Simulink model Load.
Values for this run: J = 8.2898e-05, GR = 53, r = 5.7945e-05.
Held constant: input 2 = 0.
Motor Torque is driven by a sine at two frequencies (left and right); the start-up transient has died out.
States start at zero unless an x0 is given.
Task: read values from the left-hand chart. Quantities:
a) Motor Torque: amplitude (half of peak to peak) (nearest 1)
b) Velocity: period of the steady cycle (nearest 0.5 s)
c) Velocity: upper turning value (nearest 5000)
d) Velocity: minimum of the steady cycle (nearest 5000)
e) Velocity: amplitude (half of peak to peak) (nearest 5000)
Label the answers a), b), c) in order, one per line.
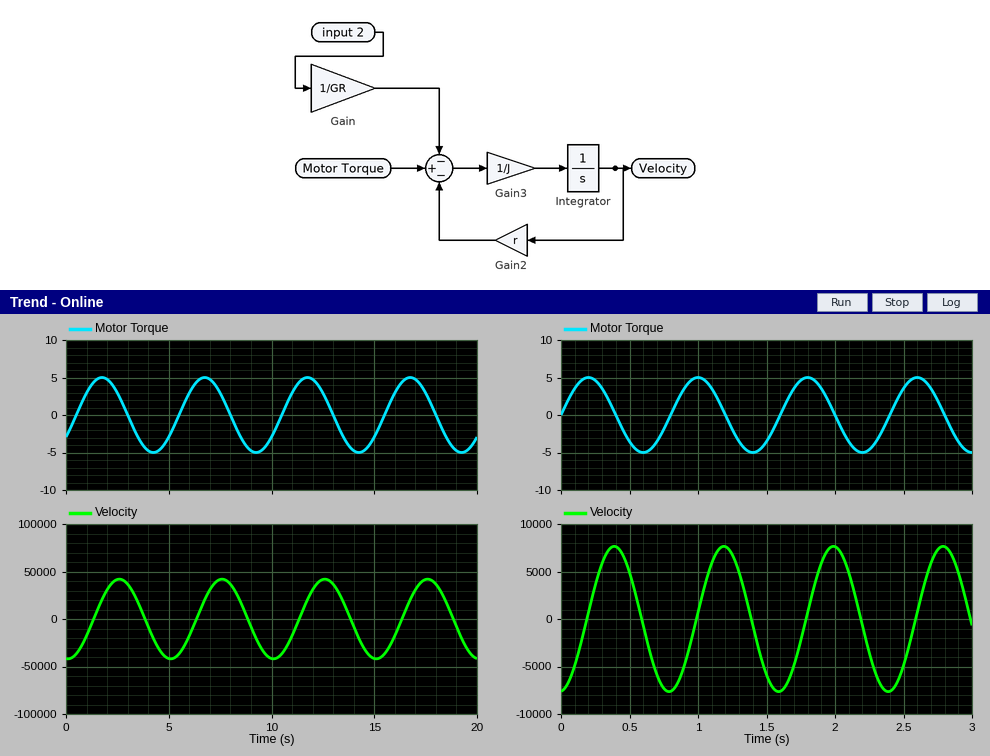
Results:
a) 5
b) 5.0 s
c) 40000
d) -40000
e) 40000
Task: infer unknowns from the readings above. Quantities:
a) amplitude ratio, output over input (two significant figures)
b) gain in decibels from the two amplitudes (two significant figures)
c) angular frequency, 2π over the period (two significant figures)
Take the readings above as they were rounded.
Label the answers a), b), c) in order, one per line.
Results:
a) 8000
b) 78 dB
c) 1.3 rad/s
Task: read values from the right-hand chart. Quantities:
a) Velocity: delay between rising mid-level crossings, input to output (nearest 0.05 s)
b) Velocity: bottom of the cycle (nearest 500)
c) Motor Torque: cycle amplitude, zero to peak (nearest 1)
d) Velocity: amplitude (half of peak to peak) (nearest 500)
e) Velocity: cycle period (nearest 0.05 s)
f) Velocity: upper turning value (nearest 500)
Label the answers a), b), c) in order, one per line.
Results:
a) 0.20 s
b) -7500
c) 5
d) 7500
e) 0.80 s
f) 7500
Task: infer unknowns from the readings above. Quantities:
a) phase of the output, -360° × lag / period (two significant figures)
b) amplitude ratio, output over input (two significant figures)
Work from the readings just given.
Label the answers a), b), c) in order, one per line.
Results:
a) -90°
b) 1500
